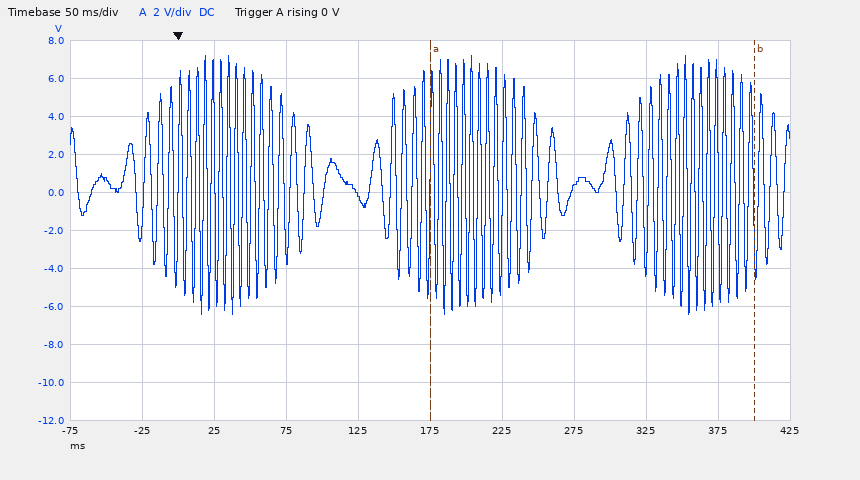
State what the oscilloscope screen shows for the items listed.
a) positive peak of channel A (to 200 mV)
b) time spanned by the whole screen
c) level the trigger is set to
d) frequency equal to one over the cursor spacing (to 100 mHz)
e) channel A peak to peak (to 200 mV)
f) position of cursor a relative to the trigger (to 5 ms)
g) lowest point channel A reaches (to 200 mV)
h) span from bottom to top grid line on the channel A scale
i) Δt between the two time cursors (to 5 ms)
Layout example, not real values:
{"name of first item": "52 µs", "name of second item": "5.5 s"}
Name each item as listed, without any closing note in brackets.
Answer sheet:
{"positive peak of channel A": "7.2 V", "time spanned by the whole screen": "500 ms", "level the trigger is set to": "0 V", "frequency equal to one over the cursor spacing": "4.4 Hz", "channel A peak to peak": "13.6 V", "position of cursor a relative to the trigger": "+175 ms", "lowest point channel A reaches": "-6.4 V", "span from bottom to top grid line on the channel A scale": "20 V", "Δt between the two time cursors": "225 ms"}
